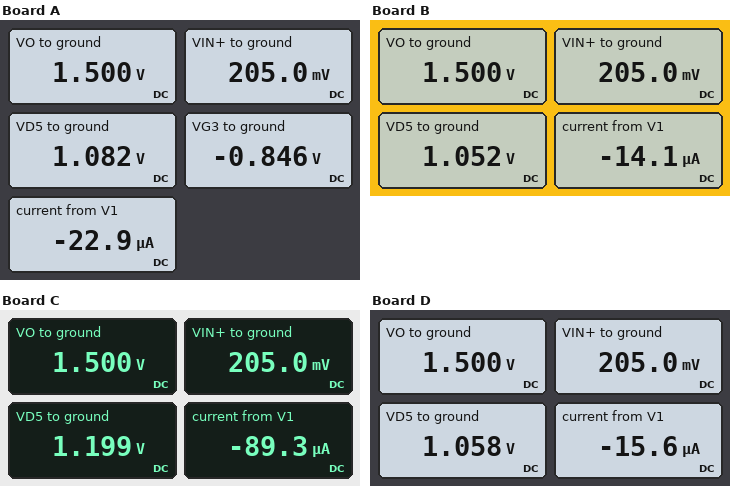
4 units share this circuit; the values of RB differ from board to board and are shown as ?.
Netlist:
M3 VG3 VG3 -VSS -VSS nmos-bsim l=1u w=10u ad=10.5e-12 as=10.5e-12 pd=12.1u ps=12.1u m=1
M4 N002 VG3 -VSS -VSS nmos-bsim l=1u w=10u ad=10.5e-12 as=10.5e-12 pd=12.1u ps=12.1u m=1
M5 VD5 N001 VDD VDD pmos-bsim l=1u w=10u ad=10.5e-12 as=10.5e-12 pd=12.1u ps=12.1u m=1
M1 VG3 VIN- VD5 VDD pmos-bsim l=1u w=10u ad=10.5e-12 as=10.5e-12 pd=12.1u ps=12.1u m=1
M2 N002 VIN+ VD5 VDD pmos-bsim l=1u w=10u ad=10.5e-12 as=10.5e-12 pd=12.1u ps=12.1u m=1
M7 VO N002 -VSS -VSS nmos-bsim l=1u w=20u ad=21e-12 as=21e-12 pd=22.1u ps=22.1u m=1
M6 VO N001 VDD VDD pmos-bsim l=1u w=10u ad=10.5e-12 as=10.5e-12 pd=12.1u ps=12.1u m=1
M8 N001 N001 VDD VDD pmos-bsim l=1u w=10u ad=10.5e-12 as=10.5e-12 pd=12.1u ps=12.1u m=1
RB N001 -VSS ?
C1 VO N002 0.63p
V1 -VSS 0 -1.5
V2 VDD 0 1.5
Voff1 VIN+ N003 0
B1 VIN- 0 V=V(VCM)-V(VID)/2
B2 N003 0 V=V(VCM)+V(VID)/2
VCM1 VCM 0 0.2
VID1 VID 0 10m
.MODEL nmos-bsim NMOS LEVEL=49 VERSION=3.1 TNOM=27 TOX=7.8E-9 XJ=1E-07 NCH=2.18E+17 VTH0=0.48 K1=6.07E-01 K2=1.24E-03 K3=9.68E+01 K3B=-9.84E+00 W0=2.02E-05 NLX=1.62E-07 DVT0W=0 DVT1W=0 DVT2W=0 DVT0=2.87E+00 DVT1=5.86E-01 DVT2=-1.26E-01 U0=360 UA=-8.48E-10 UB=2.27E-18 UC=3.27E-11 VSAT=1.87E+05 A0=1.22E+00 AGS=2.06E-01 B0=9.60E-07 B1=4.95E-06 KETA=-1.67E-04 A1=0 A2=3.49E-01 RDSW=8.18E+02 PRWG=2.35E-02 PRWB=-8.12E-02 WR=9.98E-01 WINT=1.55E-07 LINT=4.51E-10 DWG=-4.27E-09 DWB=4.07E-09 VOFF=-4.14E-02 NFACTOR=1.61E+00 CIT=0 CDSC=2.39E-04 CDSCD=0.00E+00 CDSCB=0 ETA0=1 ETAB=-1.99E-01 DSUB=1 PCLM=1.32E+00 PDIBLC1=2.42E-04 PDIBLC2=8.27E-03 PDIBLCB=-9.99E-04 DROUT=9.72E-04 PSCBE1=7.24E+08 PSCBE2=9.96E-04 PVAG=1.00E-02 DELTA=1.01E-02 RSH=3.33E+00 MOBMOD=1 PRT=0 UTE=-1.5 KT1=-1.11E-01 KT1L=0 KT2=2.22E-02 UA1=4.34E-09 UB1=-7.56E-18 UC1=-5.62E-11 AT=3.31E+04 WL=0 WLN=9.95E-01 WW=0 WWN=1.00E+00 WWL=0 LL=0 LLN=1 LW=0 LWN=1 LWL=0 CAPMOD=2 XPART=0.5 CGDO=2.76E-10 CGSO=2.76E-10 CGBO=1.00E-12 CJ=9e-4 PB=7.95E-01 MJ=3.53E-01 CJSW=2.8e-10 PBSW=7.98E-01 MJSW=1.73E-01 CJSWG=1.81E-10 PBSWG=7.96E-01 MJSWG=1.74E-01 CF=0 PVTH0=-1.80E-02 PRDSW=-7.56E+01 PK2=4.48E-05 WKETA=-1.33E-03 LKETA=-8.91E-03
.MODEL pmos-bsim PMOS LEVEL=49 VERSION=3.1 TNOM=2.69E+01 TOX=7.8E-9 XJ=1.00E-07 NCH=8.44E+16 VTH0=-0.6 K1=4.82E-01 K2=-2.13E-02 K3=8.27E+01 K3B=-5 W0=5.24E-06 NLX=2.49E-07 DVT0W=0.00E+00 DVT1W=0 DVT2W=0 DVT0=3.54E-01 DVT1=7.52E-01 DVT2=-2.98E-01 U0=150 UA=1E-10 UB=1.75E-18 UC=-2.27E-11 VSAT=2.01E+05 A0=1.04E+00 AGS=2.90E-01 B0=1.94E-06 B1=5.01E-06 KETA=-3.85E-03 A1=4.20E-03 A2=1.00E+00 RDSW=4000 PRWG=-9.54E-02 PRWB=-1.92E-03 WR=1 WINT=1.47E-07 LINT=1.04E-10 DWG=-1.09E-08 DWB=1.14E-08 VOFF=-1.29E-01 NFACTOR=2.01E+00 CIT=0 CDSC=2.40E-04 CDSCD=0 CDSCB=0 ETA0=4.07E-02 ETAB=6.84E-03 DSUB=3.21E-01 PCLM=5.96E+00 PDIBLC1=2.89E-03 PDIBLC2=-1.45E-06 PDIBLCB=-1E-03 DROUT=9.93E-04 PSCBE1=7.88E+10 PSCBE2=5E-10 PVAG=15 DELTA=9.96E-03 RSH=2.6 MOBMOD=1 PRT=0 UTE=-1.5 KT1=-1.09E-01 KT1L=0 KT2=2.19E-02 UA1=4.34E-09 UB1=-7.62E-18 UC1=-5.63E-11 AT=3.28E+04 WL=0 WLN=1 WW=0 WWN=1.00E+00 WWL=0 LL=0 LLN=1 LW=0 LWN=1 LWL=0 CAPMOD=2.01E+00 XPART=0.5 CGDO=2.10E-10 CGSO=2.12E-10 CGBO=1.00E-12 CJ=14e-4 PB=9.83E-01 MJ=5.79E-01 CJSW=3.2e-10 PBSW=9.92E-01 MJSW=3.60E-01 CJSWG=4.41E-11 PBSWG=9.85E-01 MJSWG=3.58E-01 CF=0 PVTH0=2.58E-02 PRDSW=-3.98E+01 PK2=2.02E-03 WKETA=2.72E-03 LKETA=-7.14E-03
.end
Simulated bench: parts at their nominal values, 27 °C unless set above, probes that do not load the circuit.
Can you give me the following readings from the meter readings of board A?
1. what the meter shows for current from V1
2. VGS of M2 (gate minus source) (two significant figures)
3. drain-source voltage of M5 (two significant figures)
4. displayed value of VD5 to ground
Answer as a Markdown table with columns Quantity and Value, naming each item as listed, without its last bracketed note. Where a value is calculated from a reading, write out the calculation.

| Quantity | Value |
|---|---|
| what the meter shows for current from V1 | -22.9 µA |
| VGS of M2 (gate minus source) | 205 mV - 1.082 V = -880 mV |
| drain-source voltage of M5 | 1.082 V - 1.5 V = -420 mV |
| displayed value of VD5 to ground | 1.082 V |
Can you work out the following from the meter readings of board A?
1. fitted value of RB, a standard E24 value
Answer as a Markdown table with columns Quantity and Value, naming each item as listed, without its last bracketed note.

| Quantity | Value |
|---|---|
| fitted value of RB, a standard E24 value | 180 kΩ |
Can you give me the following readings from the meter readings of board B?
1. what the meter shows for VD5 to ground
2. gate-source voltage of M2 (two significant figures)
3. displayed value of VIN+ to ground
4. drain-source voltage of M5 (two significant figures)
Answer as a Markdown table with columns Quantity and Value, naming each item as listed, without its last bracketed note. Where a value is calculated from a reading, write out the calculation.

| Quantity | Value |
|---|---|
| what the meter shows for VD5 to ground | 1.052 V |
| gate-source voltage of M2 | 205 mV - 1.052 V = -850 mV |
| displayed value of VIN+ to ground | 205.0 mV |
| drain-source voltage of M5 | 1.052 V - 1.5 V = -450 mV |
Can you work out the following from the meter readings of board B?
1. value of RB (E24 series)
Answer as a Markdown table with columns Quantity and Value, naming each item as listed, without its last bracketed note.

| Quantity | Value |
|---|---|
| value of RB | 300 kΩ |
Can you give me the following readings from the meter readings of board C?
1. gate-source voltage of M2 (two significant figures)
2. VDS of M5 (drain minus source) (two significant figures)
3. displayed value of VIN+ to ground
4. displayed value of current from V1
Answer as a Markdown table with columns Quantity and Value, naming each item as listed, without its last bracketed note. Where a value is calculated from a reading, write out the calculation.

| Quantity | Value |
|---|---|
| gate-source voltage of M2 | 205 mV - 1.199 V = -990 mV |
| VDS of M5 (drain minus source) | 1.199 V - 1.5 V = -300 mV |
| displayed value of VIN+ to ground | 205.0 mV |
| displayed value of current from V1 | -89.3 µA |
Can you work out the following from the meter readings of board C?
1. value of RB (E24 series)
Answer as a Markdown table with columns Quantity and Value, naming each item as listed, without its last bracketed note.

| Quantity | Value |
|---|---|
| value of RB | 39 kΩ |
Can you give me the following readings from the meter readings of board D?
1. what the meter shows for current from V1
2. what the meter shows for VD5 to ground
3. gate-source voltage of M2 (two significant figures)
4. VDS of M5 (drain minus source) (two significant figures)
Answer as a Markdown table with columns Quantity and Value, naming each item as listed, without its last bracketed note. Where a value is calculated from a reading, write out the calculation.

| Quantity | Value |
|---|---|
| what the meter shows for current from V1 | -15.6 µA |
| what the meter shows for VD5 to ground | 1.058 V |
| gate-source voltage of M2 | 205 mV - 1.058 V = -850 mV |
| VDS of M5 (drain minus source) | 1.058 V - 1.5 V = -440 mV |
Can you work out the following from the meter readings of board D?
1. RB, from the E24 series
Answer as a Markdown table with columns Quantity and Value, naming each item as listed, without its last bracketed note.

| Quantity | Value |
|---|---|
| RB, from the E24 series | 270 kΩ |
